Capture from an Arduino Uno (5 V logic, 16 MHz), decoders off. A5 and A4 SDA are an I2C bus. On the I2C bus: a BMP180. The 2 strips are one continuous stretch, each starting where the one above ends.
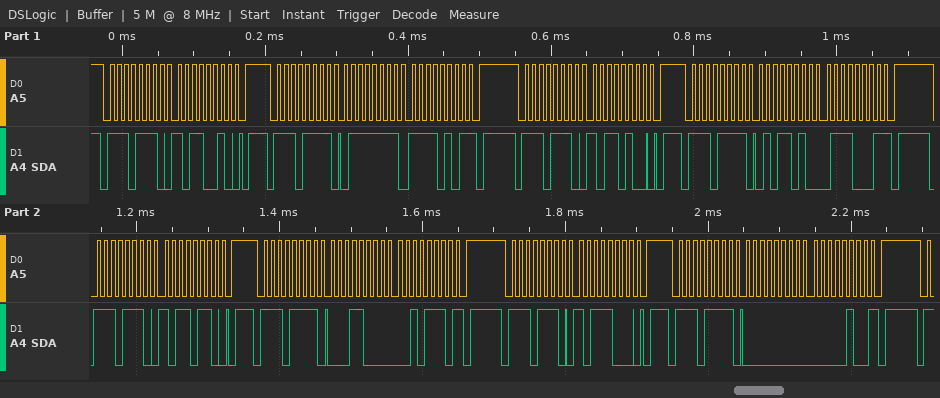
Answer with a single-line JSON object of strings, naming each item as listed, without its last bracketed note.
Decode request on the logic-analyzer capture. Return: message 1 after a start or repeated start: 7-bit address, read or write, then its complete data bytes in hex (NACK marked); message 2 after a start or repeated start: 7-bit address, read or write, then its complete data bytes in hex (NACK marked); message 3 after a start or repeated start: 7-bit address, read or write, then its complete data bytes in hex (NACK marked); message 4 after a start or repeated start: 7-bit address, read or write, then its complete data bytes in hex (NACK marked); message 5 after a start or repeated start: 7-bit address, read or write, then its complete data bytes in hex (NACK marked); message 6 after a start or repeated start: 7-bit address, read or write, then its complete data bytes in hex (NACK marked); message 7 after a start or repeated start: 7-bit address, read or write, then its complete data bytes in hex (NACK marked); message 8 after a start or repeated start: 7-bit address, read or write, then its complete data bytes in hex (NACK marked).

{"message 1 after a start or repeated start: 7-bit address, read or write, then its complete data bytes in hex": "0x77 write: B2", "message 2 after a start or repeated start: 7-bit address, read or write, then its complete data bytes in hex": "0x77 read: 7F F5 NACK", "message 3 after a start or repeated start: 7-bit address, read or write, then its complete data bytes in hex": "0x77 write: B4", "message 4 after a start or repeated start: 7-bit address, read or write, then its complete data bytes in hex": "0x77 read: 5A 71 NACK", "message 5 after a start or repeated start: 7-bit address, read or write, then its complete data bytes in hex": "0x77 write: B6", "message 6 after a start or repeated start: 7-bit address, read or write, then its complete data bytes in hex": "0x77 read: 18 2E NACK", "message 7 after a start or repeated start: 7-bit address, read or write, then its complete data bytes in hex": "0x77 write: B8", "message 8 after a start or repeated start: 7-bit address, read or write, then its complete data bytes in hex": "0x77 read: 00 04 NACK"}
